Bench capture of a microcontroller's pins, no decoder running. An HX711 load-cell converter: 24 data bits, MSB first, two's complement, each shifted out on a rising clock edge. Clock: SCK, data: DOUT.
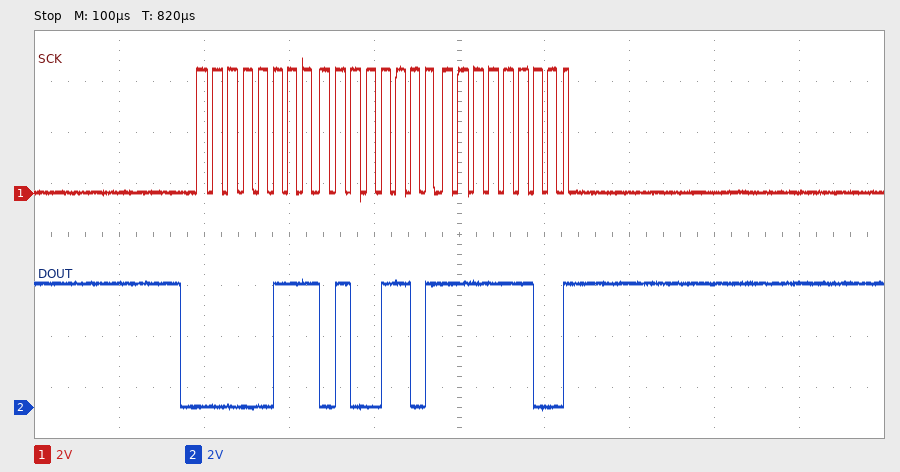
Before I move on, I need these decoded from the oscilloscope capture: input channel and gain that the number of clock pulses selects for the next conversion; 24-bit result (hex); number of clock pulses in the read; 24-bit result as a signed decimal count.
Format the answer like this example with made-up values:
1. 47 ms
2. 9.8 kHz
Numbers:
1. channel A, gain 128
2. 0x074DFC
3. 25
4. 478716
